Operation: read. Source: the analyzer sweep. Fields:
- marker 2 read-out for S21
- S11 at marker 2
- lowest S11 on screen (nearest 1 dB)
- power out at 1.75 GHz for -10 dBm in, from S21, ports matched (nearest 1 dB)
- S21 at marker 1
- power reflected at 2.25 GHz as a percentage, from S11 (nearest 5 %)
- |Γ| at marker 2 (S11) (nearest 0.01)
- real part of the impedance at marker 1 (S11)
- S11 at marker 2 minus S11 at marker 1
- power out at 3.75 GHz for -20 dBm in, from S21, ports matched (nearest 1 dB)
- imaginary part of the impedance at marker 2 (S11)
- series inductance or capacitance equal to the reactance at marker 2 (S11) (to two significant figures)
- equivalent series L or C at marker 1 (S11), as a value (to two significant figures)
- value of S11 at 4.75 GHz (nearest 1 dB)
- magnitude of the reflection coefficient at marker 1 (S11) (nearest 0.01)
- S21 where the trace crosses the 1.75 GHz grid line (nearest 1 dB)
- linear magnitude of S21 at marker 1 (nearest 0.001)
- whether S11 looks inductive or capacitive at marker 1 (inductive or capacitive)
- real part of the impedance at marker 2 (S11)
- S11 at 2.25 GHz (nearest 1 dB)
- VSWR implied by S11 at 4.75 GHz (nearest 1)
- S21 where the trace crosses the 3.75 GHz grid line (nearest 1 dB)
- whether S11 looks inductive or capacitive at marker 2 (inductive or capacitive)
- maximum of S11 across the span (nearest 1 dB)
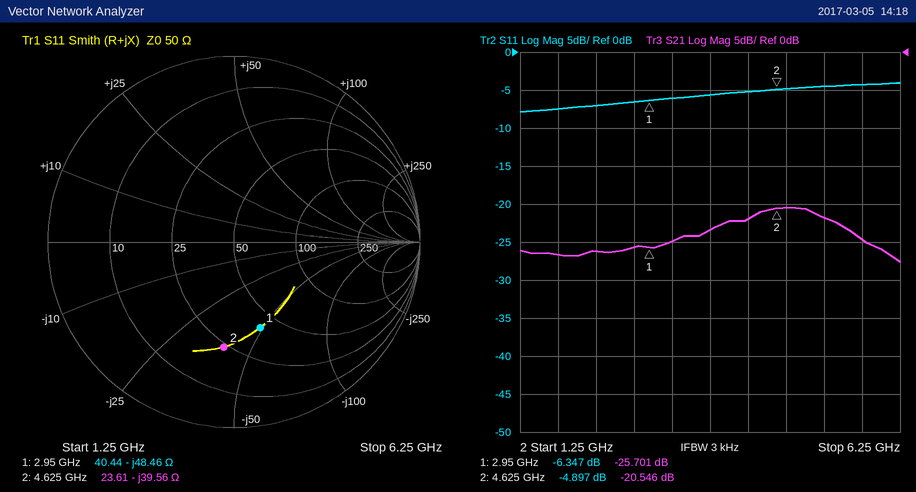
-20.546 dB
-4.897 dB
-8 dB
-37 dBm
-25.701 dB
20 %
0.57
40.44 Ω
1.450 dB
-43 dBm
-39.56 Ω
870 fF
1.1 pF
-5 dB
0.48
-27 dB
0.052
capacitive
23.61 Ω
-7 dB
4
-23 dB
capacitive
-4 dB
